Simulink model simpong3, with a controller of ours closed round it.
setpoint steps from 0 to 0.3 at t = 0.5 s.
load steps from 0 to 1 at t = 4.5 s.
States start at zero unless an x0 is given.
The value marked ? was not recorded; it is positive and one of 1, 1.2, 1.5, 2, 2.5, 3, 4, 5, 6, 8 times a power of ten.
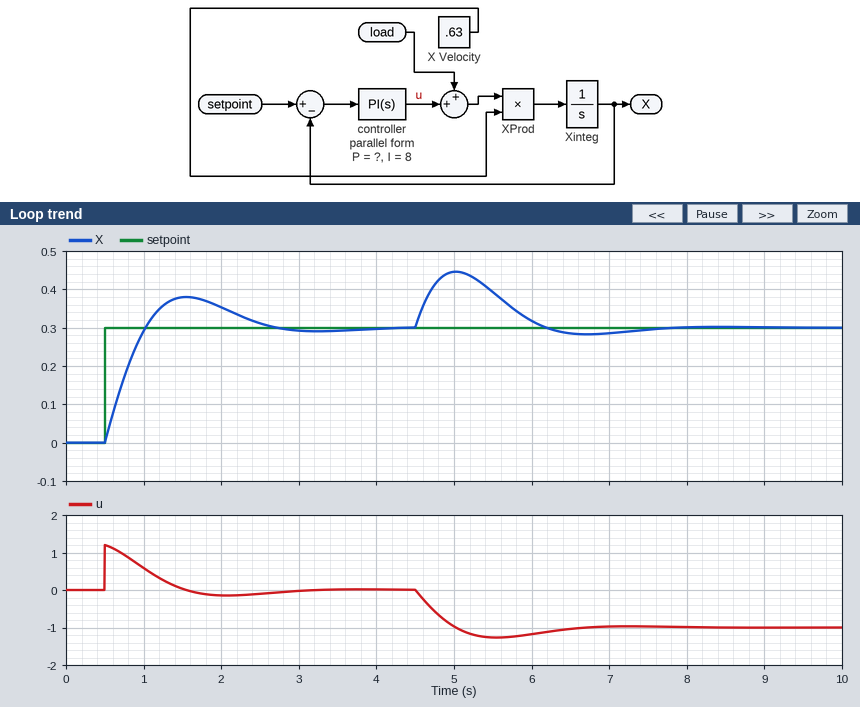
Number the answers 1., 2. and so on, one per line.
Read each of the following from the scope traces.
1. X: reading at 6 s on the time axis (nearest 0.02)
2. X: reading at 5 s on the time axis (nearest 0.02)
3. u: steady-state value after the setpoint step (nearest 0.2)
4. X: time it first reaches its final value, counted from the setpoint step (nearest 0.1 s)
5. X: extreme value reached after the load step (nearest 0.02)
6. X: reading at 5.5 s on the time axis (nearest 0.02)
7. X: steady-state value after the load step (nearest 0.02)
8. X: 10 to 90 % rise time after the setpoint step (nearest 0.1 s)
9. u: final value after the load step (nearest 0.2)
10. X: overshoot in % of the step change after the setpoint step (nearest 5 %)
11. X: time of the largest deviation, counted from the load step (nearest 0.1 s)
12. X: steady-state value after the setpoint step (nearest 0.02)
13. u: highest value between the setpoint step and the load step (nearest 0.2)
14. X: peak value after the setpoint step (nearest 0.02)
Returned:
1. 0.32
2. 0.44
3. 0.0
4. 0.5 s
5. 0.44
6. 0.40
7. 0.30
8. 0.4 s
9. -1.0
10. 25 %
11. 0.5 s
12. 0.30
13. 1.2
14. 0.38
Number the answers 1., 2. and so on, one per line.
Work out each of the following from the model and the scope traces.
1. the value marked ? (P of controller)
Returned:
1. 4
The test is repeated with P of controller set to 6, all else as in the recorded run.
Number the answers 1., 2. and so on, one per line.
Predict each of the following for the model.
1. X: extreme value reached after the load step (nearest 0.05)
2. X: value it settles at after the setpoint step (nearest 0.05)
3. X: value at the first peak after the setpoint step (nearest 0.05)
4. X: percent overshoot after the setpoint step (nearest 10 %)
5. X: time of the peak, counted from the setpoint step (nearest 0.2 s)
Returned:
1. 0.40
2. 0.30
3. 0.35
4. 20 %
5. 1.0 s
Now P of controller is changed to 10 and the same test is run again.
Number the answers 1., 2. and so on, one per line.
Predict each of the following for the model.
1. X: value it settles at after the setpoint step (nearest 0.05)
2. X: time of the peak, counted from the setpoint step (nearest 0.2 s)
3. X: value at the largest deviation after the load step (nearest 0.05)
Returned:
1. 0.30
2. 0.8 s
3. 0.40
